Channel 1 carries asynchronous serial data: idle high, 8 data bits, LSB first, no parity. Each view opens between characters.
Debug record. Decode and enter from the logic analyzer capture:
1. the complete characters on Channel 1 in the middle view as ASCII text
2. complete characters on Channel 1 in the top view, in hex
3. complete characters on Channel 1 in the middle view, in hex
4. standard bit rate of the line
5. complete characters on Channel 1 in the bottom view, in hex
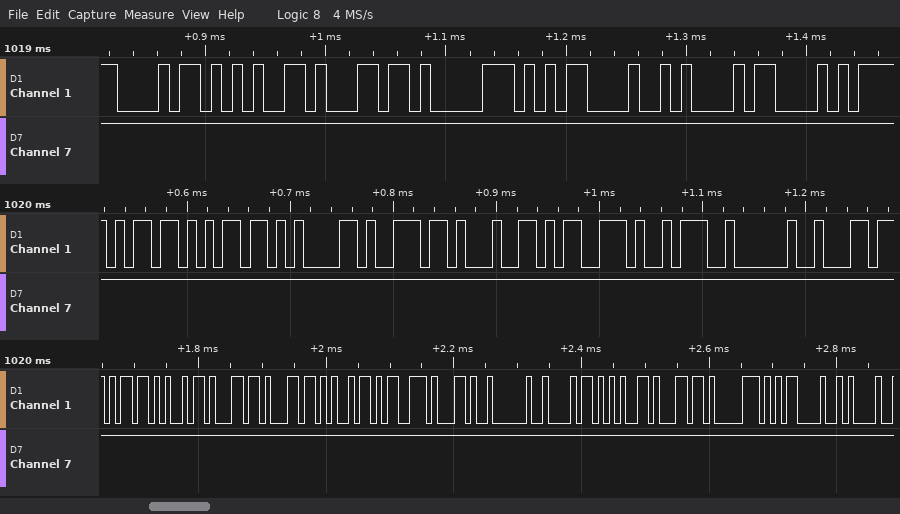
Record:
"mmands: "
68, 65, 6C, 70, 0D, 0A, 43
6D, 6D, 61, 6E, 64, 73, 3A, 20
115200 baud
6D, 69, 6C, 6C, 69, 73, 2C, 20, 68, 65, 6C, 70, 0D, 0A
